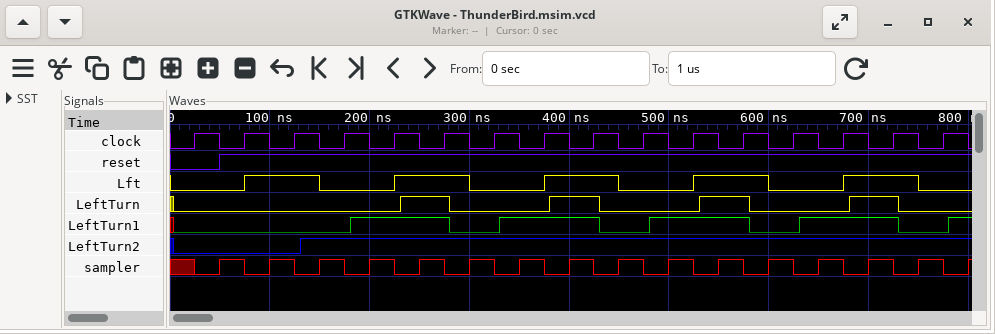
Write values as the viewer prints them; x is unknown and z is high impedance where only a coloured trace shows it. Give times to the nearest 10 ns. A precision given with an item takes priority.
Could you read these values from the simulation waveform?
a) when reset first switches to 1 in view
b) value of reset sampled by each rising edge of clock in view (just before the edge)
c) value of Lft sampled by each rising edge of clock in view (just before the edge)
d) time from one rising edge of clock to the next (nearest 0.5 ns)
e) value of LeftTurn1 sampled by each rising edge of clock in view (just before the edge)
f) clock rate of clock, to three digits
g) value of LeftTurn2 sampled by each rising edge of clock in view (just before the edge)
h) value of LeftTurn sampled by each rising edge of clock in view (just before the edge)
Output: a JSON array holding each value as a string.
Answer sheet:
["50 ns", "0 1 1 1 1 1 1 1 1 1 1 1 1 1 1 1", "0 0 1 0 0 1 0 0 1 0 0 1 0 0 1 0", "50 ns", "0 0 0 0 1 1 0 1 1 0 1 1 0 1 1 0", "20.0 MHz", "0 0 0 1 1 1 1 1 1 1 1 1 1 1 1 1", "0 0 0 0 0 1 0 0 1 0 0 1 0 0 1 0"]
